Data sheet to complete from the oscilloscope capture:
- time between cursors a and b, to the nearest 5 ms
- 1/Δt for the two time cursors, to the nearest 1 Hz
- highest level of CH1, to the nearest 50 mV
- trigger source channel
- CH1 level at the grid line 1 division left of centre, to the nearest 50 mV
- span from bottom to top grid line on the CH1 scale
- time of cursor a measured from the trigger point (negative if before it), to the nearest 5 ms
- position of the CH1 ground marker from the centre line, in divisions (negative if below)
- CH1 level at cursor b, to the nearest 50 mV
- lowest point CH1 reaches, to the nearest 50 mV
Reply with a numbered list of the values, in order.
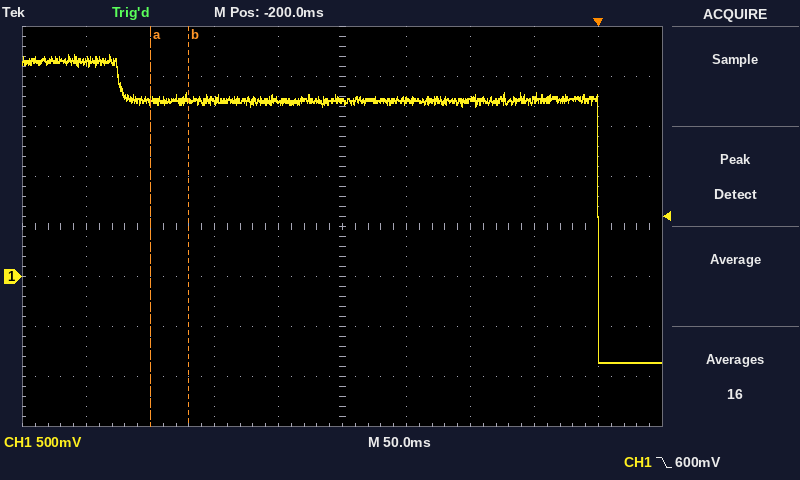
1. 30 ms
2. 33 Hz
3. 2.20 V
4. CH1
5. 1.75 V
6. 4 V
7. -350 ms
8. -1.0 div
9. 1.80 V
10. -850 mV
